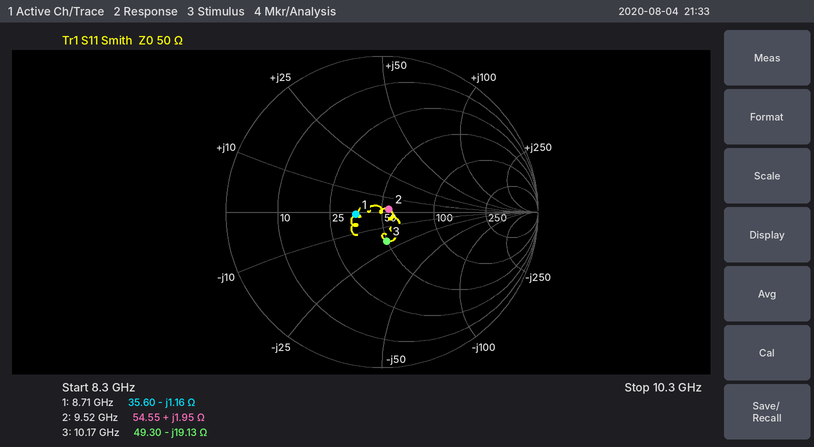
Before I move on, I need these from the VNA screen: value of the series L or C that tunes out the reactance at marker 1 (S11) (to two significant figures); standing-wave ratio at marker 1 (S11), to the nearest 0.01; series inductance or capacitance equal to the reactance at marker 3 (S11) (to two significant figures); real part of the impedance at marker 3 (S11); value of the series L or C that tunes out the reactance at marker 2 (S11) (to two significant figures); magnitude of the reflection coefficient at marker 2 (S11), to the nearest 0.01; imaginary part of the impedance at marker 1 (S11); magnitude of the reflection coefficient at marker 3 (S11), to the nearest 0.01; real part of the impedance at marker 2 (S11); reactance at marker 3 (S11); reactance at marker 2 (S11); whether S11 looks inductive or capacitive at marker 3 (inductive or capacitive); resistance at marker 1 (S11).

21 pH
1.41
820 fF
49.30 Ω
8.6 pF
0.05
-1.16 Ω
0.19
54.55 Ω
-19.13 Ω
+1.95 Ω
capacitive
35.60 Ω
